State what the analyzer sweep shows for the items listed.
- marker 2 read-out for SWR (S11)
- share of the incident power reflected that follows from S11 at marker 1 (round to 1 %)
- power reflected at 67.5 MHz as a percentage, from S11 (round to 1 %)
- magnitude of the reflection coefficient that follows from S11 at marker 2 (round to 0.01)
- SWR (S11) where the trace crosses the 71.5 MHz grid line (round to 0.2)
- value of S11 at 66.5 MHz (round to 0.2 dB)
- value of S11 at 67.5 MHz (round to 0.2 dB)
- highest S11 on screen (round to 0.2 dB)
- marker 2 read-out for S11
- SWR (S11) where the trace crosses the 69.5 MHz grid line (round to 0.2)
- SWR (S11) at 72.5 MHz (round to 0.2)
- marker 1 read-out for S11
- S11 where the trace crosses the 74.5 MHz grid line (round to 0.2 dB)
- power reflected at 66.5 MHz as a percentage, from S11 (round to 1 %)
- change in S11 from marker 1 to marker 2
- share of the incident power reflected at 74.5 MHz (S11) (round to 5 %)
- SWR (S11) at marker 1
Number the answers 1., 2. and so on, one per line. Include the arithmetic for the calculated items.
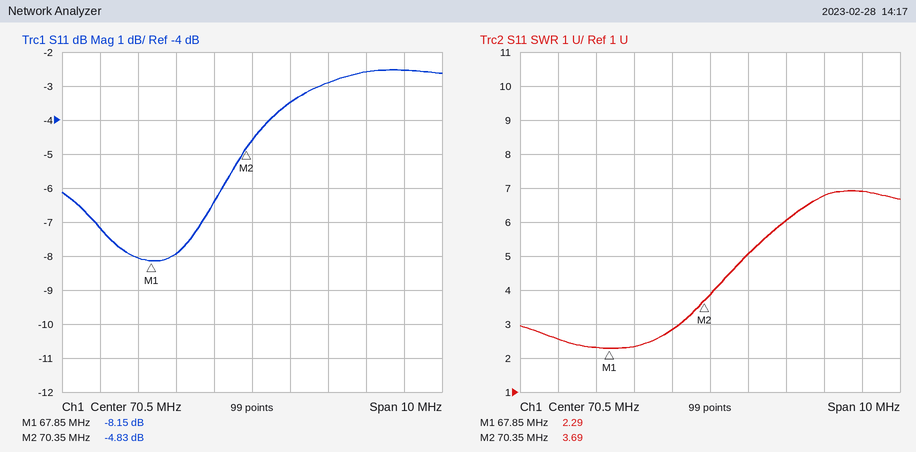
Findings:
1. 3.69
2. 10^(-8.15/10) ≈ 15 %
3. 10^(-8/10) ≈ 16 %
4. 10^(-4.83/20) ≈ 0.57
5. 5.0
6. -7.2 dB
7. -8.0 dB
8. -2.6 dB
9. -4.83 dB
10. 2.8
11. 6.0
12. -8.15 dB
13. -2.6 dB
14. 10^(-7.2/10) ≈ 19 %
15. -4.83 − (-8.15) = 3.32 dB
16. 10^(-2.6/10) ≈ 55 %
17. 2.29
